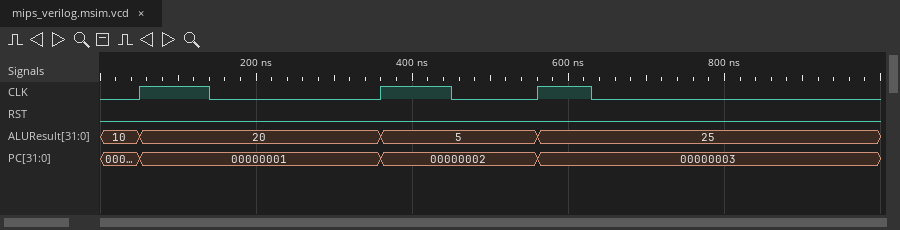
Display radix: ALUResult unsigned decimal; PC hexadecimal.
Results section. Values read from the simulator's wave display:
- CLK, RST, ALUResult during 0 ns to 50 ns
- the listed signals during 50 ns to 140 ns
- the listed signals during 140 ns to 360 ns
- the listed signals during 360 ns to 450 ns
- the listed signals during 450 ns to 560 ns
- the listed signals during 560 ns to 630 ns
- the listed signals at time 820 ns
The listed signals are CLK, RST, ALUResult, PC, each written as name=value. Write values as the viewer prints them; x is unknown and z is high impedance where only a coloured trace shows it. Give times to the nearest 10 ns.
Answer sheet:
CLK=0, RST=0, ALUResult=10
CLK=1, RST=0, ALUResult=20, PC=00000001
CLK=0, RST=0, ALUResult=20, PC=00000001
CLK=1, RST=0, ALUResult=5, PC=00000002
CLK=0, RST=0, ALUResult=5, PC=00000002
CLK=1, RST=0, ALUResult=25, PC=00000003
CLK=0, RST=0, ALUResult=25, PC=00000003
